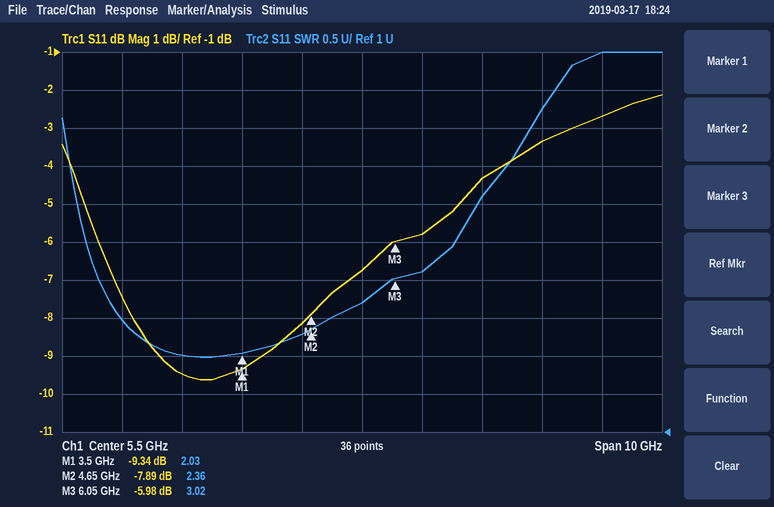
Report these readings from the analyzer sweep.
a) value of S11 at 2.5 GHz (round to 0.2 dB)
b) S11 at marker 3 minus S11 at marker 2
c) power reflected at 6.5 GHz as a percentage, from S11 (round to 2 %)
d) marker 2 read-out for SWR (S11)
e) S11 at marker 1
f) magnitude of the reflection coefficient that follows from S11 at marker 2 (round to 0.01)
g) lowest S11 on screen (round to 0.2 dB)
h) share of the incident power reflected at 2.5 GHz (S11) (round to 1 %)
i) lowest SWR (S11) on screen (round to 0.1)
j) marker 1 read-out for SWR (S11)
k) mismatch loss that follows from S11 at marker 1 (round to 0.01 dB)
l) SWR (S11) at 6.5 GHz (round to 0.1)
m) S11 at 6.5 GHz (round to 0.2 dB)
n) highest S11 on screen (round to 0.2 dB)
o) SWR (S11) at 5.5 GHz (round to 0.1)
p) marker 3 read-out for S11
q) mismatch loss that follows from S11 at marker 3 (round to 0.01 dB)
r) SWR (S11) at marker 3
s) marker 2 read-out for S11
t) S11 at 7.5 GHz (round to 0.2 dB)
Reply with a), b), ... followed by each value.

a) -9.4 dB
b) 1.91 dB
c) 26 %
d) 2.36
e) -9.34 dB
f) 0.40
g) -9.6 dB
h) 11 %
i) 2.0
j) 2.03
k) 0.54 dB
l) 3.1
m) -5.8 dB
n) -2.2 dB
o) 2.7
p) -5.98 dB
q) 1.26 dB
r) 3.02
s) -7.89 dB
t) -4.4 dB
